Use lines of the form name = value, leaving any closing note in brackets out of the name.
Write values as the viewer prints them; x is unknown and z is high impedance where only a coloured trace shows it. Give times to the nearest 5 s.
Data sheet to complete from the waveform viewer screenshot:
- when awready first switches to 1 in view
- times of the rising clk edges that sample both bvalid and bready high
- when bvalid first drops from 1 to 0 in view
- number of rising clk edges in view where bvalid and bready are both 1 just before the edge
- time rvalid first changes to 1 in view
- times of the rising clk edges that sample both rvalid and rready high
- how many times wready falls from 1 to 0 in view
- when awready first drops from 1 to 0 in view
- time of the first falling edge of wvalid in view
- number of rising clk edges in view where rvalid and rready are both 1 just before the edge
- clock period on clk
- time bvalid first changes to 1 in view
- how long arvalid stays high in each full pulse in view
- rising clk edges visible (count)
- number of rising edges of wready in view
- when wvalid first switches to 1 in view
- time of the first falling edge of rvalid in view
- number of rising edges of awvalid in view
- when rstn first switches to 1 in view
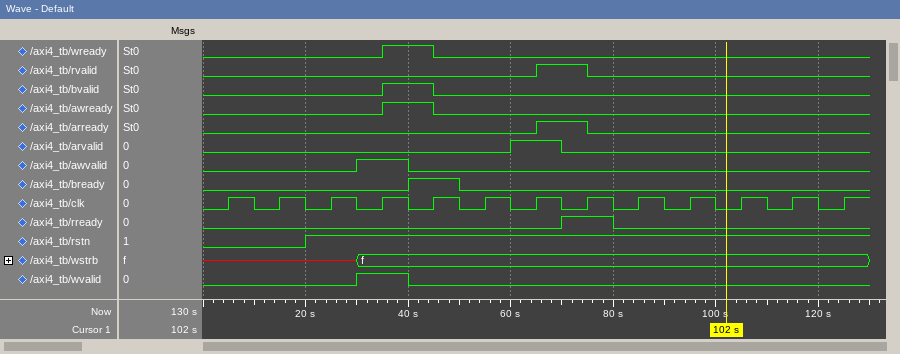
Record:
when awready first switches to 1 in view = 35 s
times of the rising clk edges that sample both bvalid and bready high = 45 s
when bvalid first drops from 1 to 0 in view = 45 s
number of rising clk edges in view where bvalid and bready are both 1 just before the edge = 1
time rvalid first changes to 1 in view = 65 s
times of the rising clk edges that sample both rvalid and rready high = 75 s
how many times wready falls from 1 to 0 in view = 1
when awready first drops from 1 to 0 in view = 45 s
time of the first falling edge of wvalid in view = 40 s
number of rising clk edges in view where rvalid and rready are both 1 just before the edge = 1
clock period on clk = 10 s
time bvalid first changes to 1 in view = 35 s
how long arvalid stays high in each full pulse in view = 10 s
rising clk edges visible = 13
number of rising edges of wready in view = 1
when wvalid first switches to 1 in view = 30 s
time of the first falling edge of rvalid in view = 75 s
number of rising edges of awvalid in view = 1
when rstn first switches to 1 in view = 20 s
